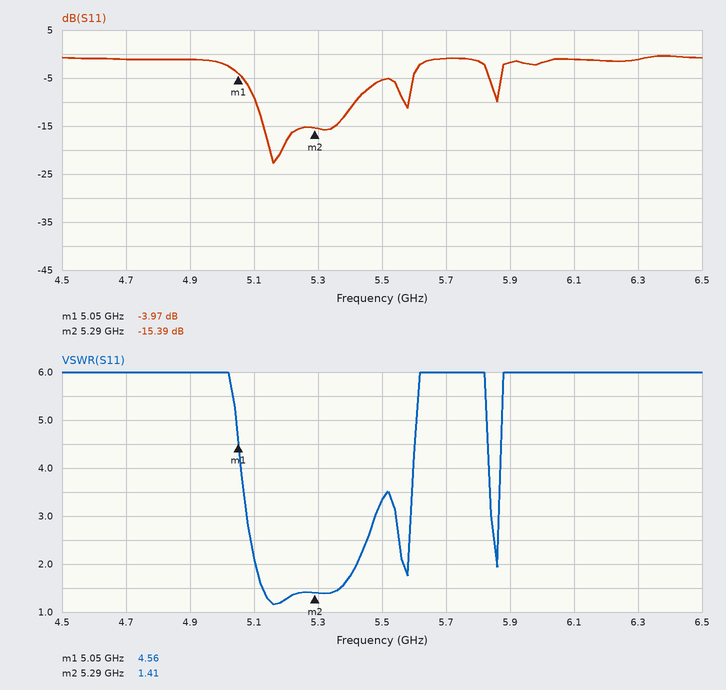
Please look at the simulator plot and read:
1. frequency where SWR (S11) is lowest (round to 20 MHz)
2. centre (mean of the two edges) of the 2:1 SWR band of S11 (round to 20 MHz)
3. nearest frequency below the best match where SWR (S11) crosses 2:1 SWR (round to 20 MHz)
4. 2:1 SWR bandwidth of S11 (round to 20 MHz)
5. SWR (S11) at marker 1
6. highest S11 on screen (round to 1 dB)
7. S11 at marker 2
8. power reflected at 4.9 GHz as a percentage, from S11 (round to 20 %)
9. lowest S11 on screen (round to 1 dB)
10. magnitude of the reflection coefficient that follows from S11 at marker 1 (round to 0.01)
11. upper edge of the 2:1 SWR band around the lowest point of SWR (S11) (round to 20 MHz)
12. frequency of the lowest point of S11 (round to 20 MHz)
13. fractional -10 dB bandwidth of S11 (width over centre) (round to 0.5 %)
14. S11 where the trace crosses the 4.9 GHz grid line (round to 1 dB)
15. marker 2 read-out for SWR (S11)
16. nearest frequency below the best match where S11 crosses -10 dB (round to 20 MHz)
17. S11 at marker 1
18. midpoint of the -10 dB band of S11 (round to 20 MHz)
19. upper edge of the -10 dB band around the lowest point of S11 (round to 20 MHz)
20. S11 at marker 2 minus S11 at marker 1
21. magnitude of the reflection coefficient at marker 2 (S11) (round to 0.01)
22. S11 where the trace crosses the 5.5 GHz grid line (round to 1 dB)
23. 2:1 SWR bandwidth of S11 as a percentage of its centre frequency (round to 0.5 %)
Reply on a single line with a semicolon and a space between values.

5.16 GHz; 5.26 GHz; 5.10 GHz; 320 MHz; 4.56; 0 dB; -15.39 dB; 80 %; -23 dB; 0.63; 5.42 GHz; 5.16 GHz; 6.0 %; -1 dB; 1.41; 5.10 GHz; -3.97 dB; 5.26 GHz; 5.42 GHz; -11.42 dB; 0.17; -5 dB; 6.0 %
